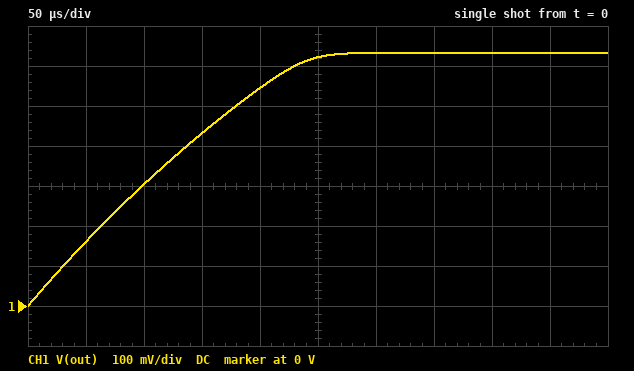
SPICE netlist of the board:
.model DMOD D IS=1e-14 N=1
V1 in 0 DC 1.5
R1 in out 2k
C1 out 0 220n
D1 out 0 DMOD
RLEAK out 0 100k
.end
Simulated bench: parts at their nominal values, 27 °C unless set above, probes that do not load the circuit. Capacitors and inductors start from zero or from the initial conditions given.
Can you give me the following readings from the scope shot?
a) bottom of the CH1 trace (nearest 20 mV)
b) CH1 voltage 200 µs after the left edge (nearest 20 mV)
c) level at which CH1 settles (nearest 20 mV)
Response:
0 V
540 mV
640 mV
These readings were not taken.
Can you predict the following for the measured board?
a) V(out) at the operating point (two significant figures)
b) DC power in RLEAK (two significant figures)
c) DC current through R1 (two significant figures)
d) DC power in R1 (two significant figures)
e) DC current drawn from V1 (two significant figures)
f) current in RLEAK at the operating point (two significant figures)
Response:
630 mV
4.0 µW
430 µA
380 µW
430 µA
6.3 µA
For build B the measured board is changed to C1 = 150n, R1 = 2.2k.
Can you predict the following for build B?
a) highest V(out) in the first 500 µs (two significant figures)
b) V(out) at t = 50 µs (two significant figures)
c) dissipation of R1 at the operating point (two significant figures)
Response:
630 mV
210 mV
340 µW
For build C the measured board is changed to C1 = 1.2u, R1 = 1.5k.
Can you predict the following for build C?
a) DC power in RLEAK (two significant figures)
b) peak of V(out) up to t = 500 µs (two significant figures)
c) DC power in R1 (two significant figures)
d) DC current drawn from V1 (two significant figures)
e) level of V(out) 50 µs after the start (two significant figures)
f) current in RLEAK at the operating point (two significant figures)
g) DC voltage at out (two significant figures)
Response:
4.1 µW
360 mV
490 µW
570 µA
41 mV
6.4 µA
640 mV
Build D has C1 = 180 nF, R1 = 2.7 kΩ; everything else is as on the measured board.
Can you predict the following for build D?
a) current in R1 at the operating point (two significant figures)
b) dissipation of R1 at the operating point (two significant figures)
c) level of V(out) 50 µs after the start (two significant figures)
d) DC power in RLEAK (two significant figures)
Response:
320 µA
280 µW
150 mV
3.9 µW
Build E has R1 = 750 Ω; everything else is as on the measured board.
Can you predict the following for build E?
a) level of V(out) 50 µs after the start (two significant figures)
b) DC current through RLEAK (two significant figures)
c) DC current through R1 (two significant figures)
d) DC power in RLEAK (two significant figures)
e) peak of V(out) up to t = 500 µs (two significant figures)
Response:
390 mV
6.6 µA
1.1 mA
4.3 µW
660 mV
